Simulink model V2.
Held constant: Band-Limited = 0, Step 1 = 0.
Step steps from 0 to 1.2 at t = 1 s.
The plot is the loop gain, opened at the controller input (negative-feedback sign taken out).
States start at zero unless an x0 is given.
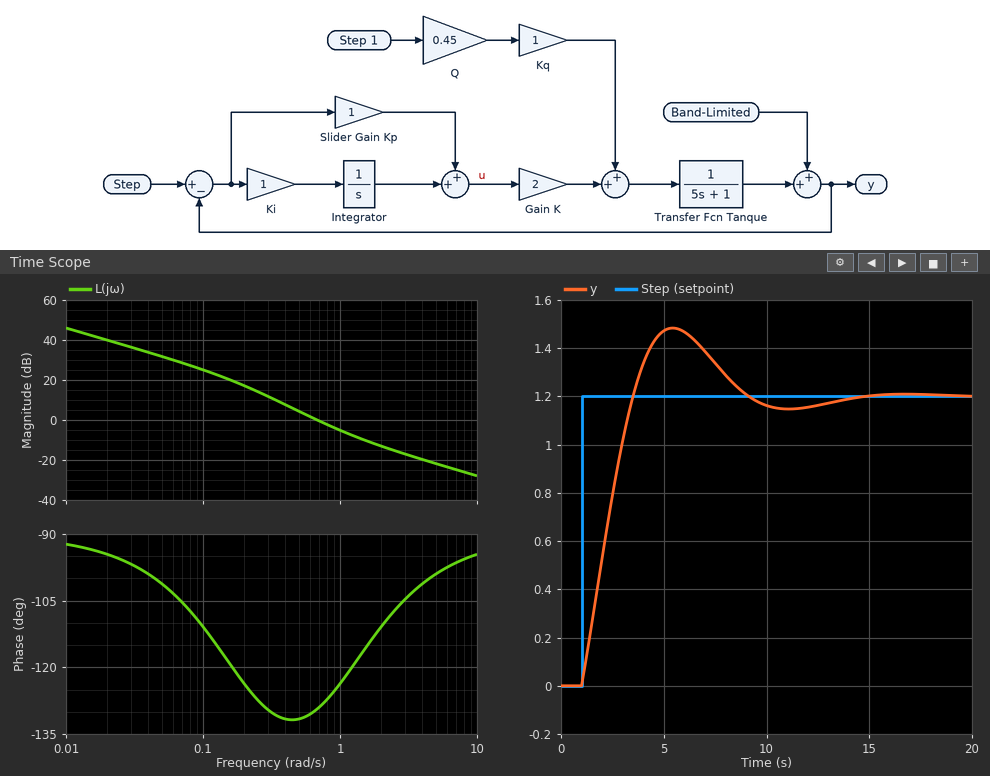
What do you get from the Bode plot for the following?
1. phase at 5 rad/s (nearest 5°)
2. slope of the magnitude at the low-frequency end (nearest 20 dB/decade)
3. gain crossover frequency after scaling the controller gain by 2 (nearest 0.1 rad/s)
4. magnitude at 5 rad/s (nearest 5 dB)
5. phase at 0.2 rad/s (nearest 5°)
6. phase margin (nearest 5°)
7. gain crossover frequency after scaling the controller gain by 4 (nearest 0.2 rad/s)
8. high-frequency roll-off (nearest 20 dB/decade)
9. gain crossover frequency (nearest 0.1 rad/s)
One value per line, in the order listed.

-100°
-20 dB/decade
1.1 rad/s
-20 dB
-125°
50°
1.8 rad/s
-20 dB/decade
0.7 rad/s
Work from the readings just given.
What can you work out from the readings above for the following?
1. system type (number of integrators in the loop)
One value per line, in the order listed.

1
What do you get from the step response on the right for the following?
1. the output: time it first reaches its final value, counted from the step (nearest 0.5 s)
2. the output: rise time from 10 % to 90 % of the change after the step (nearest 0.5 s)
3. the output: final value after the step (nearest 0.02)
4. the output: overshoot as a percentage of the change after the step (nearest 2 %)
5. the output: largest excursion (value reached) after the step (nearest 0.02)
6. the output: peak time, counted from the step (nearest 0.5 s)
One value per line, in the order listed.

2.5 s
2.0 s
1.20
24 %
1.48
4.5 s
